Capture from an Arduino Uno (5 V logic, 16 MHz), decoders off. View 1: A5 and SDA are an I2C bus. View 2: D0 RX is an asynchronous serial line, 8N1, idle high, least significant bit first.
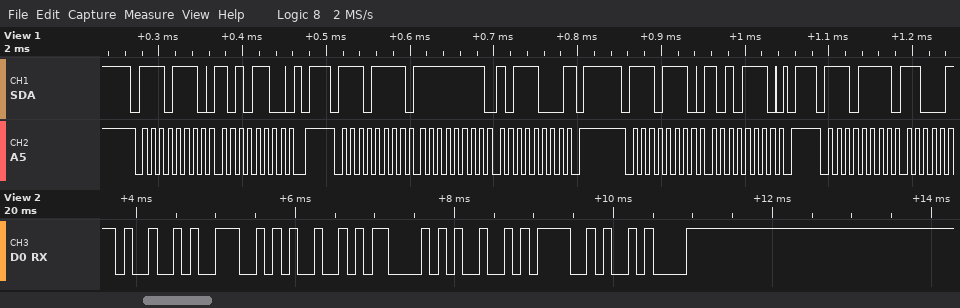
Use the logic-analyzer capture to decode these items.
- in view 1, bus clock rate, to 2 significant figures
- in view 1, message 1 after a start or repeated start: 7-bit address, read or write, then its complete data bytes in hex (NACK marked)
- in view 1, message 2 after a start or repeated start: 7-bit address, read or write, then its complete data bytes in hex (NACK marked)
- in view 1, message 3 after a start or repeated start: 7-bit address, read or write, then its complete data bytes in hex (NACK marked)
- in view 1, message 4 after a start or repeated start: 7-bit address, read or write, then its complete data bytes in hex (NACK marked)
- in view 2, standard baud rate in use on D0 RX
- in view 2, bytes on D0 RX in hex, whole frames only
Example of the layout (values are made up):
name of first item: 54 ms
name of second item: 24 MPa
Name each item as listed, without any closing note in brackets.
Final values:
in view 1, bus clock rate, to 2 significant figures: 100 kHz
in view 1, message 1 after a start or repeated start: 7-bit address, read or write, then its complete data bytes in hex: 0x77 write: AC
in view 1, message 2 after a start or repeated start: 7-bit address, read or write, then its complete data bytes in hex: 0x77 read: FF B8 NACK
in view 1, message 3 after a start or repeated start: 7-bit address, read or write, then its complete data bytes in hex: 0x77 write: AE
in view 1, message 4 after a start or repeated start: 7-bit address, read or write, then its complete data bytes in hex: 0x77 read
in view 2, standard baud rate in use on D0 RX: 9600 baud
in view 2, bytes on D0 RX in hex, whole frames only: 0x49 0x4E 0x49 0x43 0x49 0x4F 0x0A
